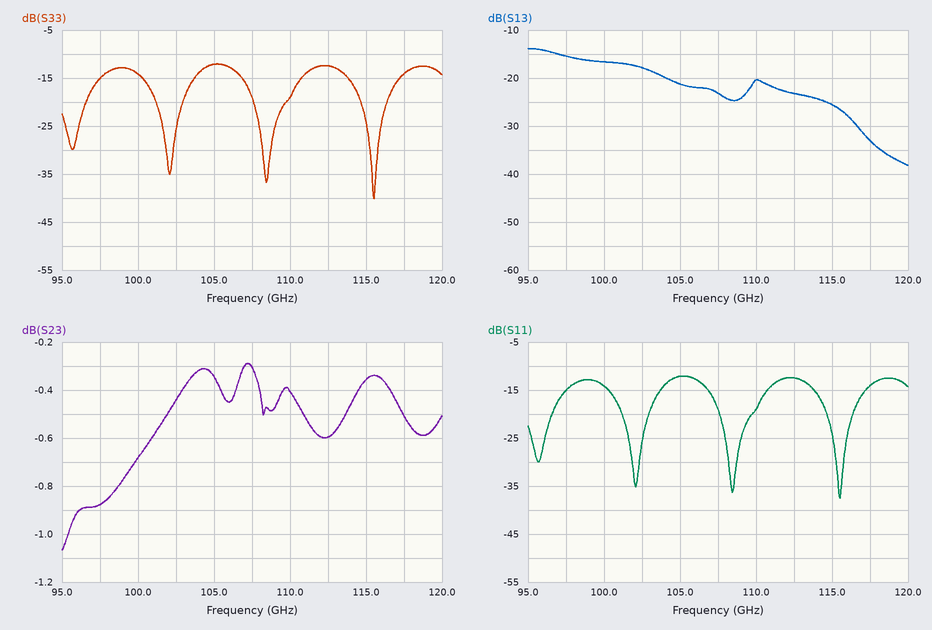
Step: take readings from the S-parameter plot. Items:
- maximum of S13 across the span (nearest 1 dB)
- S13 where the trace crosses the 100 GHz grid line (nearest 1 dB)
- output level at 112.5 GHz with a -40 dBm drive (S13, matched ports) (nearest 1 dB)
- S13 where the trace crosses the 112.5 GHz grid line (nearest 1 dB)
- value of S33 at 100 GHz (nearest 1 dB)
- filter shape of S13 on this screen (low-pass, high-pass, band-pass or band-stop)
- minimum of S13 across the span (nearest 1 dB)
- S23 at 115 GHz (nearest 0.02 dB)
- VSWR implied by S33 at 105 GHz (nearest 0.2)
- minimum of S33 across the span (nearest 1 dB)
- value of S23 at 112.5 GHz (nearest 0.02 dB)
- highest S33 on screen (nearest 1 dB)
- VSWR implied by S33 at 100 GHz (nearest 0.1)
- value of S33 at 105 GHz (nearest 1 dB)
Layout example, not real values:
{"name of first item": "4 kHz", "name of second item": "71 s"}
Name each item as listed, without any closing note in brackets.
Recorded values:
{"maximum of S13 across the span": "-14 dB", "S13 where the trace crosses the 100 GHz grid line": "-17 dB", "output level at 112.5 GHz with a -40 dBm drive (S13, matched ports)": "-63 dBm", "S13 where the trace crosses the 112.5 GHz grid line": "-23 dB", "value of S33 at 100 GHz": "-14 dB", "filter shape of S13 on this screen": "low-pass", "minimum of S13 across the span": "-38 dB", "S23 at 115 GHz": "-0.36 dB", "VSWR implied by S33 at 105 GHz": "1.6", "minimum of S33 across the span": "-40 dB", "value of S23 at 112.5 GHz": "-0.60 dB", "highest S33 on screen": "-12 dB", "VSWR implied by S33 at 100 GHz": "1.5", "value of S33 at 105 GHz": "-12 dB"}
